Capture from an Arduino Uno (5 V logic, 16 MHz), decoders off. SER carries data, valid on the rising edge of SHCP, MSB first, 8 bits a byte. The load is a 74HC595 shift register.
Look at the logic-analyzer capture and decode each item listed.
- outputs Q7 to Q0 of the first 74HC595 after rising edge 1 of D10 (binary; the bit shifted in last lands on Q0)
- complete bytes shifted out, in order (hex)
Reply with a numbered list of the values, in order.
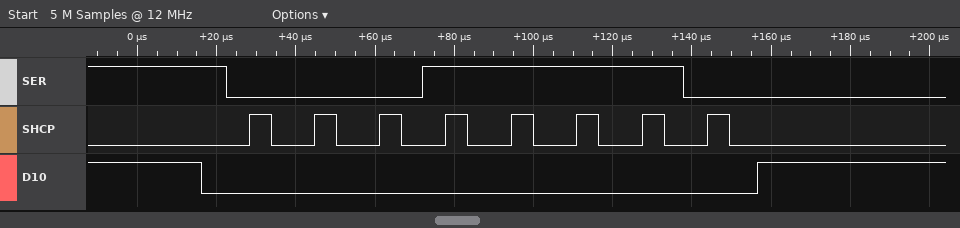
1. 00011110
2. 1E
